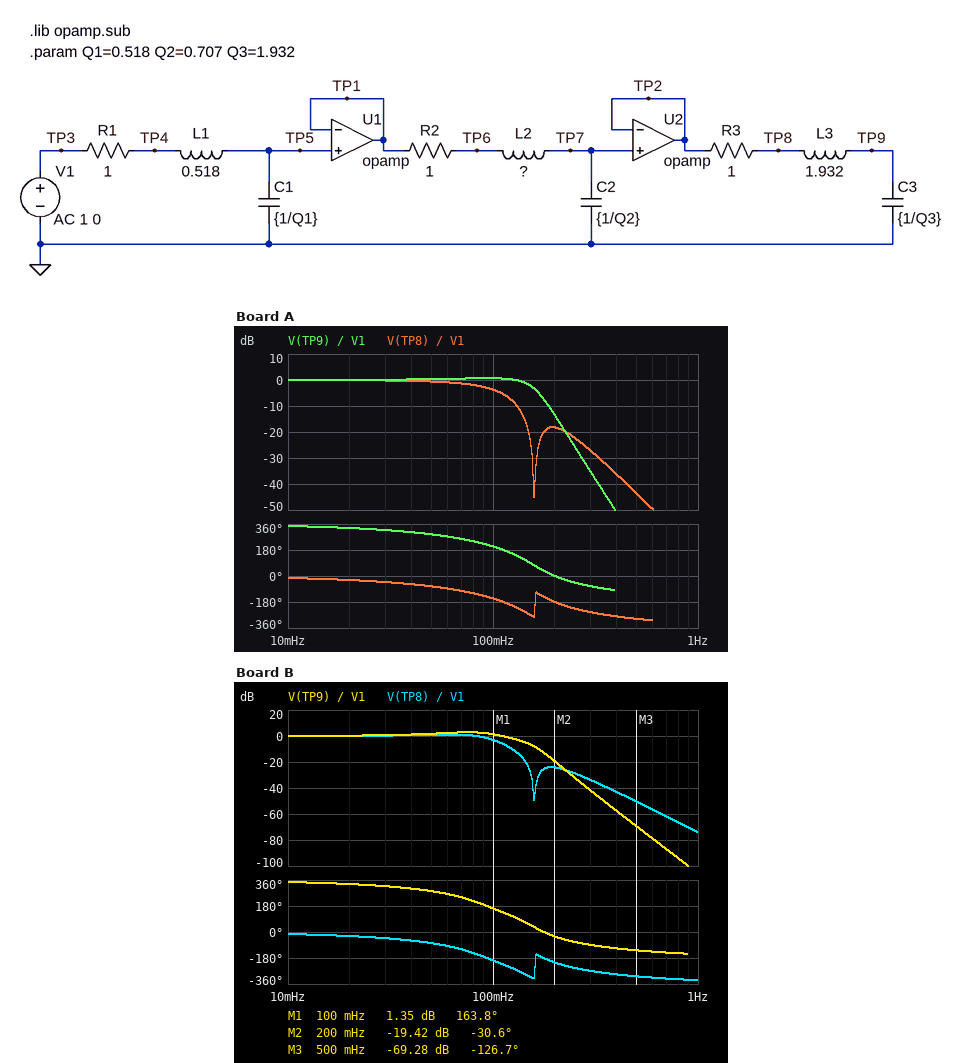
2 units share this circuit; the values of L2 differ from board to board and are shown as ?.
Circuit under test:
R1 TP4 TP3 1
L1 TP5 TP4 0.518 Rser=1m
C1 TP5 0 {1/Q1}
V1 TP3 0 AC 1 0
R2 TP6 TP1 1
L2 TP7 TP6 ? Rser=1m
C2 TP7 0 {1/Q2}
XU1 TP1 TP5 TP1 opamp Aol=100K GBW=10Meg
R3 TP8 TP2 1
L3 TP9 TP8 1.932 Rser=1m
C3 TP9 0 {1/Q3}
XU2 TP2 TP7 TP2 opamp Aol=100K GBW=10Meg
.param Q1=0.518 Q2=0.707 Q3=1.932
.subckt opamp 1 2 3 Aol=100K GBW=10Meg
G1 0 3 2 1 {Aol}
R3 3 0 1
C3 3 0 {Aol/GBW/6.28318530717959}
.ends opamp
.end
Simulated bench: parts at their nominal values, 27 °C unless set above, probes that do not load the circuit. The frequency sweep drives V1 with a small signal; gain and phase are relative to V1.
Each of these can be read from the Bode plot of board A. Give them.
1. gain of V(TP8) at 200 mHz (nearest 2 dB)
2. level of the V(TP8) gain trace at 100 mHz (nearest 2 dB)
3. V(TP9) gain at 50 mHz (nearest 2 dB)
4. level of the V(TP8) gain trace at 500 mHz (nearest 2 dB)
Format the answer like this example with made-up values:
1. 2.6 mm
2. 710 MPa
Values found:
1. -18 dB
2. -4 dB
3. 0 dB
4. -44 dB
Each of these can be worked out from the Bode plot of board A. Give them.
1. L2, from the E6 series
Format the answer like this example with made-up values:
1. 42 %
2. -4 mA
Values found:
1. 1 H
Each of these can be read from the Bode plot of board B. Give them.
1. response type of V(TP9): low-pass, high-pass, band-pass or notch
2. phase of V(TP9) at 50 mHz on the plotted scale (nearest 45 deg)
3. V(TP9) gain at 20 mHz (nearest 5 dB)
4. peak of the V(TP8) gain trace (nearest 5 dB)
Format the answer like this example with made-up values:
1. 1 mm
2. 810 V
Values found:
1. low-pass
2. 270 deg
3. 0 dB
4. 0 dB
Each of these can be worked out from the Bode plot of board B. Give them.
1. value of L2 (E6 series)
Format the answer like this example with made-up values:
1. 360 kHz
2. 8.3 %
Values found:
1. 2.2 H
